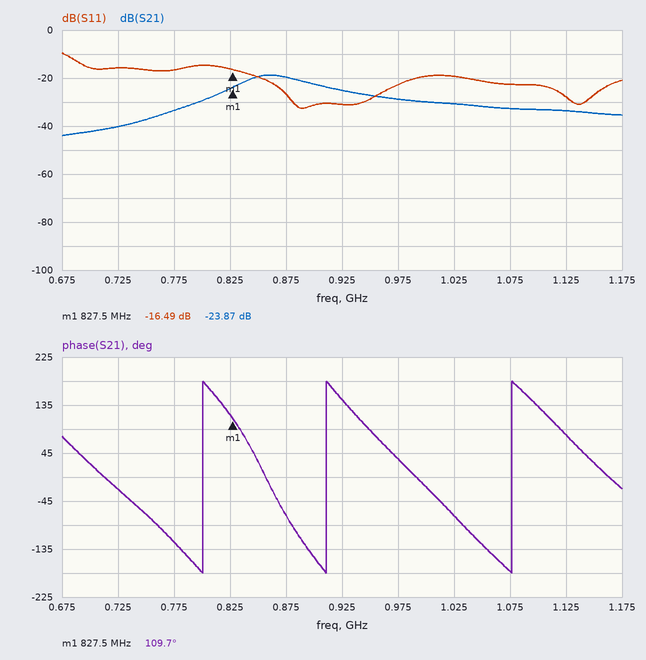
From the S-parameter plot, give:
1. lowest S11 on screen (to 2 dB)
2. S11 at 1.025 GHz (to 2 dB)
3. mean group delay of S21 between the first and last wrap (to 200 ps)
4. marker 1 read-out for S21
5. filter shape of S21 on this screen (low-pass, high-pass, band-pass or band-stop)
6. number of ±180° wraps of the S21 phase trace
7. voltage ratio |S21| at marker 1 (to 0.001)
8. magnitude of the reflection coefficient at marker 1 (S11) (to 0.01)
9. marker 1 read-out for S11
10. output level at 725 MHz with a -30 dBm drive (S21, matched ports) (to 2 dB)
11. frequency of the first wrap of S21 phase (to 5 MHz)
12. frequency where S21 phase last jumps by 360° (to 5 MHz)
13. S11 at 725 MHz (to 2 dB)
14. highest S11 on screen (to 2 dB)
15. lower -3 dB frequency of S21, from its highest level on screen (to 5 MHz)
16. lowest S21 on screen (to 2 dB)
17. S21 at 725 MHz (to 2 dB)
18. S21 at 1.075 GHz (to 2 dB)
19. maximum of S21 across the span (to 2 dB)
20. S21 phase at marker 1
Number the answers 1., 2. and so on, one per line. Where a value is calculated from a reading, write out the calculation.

1. -32 dB
2. -20 dB
3. 2 cycles / (1.075 GHz − 800 MHz) ≈ 7.27 ns, so 7.2 ns to the nearest 200 ps
4. -23.87 dB
5. band-pass
6. 3
7. 10^(-23.87/20) ≈ 0.064
8. 10^(-16.49/20) ≈ 0.15
9. -16.49 dB
10. -30 dBm + (-40 dB) = -70 dBm
11. 800 MHz
12. 1.075 GHz
13. -16 dB
14. -10 dB
15. 835 MHz
16. -44 dB
17. -40 dB
18. -32 dB
19. -18 dB
20. 109.7°
